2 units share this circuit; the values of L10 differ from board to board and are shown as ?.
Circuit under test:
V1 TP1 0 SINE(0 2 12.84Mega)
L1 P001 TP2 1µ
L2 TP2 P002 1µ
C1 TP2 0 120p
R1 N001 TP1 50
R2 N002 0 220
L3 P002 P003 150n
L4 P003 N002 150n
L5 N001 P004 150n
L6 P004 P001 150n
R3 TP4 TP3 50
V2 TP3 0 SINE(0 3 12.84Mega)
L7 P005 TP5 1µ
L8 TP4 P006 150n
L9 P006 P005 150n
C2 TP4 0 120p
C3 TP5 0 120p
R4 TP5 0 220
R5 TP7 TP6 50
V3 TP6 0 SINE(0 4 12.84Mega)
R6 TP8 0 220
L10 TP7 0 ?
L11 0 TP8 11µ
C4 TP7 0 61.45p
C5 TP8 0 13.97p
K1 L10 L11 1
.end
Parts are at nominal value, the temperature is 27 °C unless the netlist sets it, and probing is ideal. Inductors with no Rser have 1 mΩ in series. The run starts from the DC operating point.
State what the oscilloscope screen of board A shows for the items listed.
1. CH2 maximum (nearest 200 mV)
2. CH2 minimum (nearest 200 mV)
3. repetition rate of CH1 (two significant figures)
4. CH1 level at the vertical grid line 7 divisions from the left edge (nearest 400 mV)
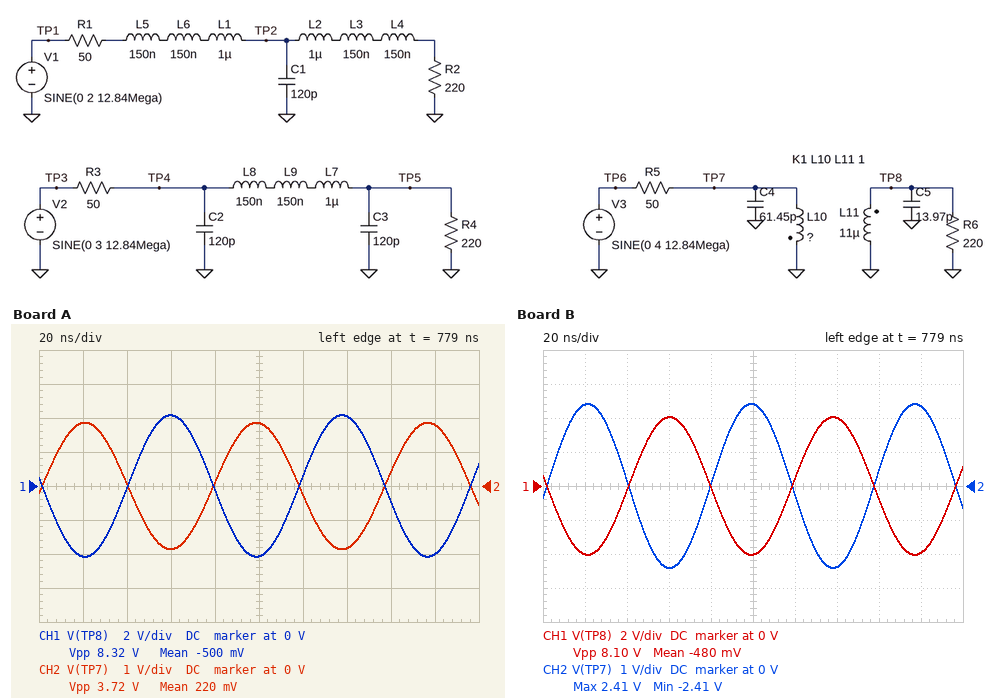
1.8 V
-1.8 V
13 MHz
4.0 V
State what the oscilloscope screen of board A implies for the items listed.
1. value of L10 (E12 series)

2.2 µH
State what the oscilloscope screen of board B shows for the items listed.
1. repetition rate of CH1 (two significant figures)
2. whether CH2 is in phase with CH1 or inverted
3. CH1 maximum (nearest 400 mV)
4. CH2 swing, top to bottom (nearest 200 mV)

13 MHz
inverted
4.0 V
4.8 V
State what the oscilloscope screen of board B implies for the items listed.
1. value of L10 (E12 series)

3.9 µH
